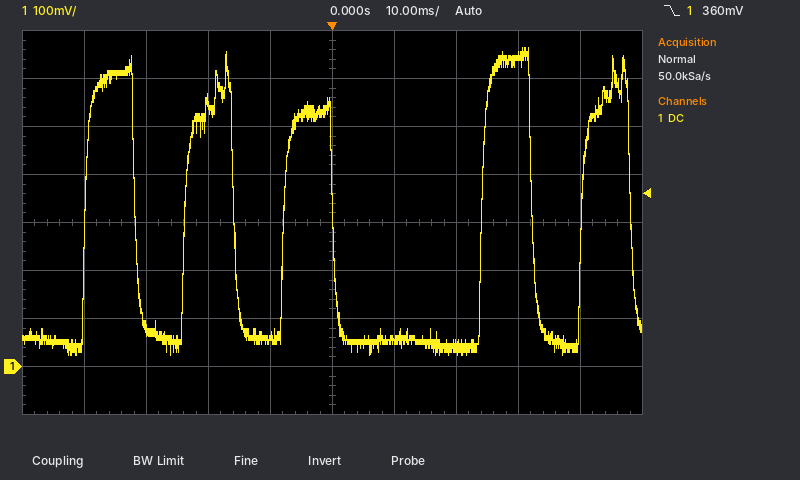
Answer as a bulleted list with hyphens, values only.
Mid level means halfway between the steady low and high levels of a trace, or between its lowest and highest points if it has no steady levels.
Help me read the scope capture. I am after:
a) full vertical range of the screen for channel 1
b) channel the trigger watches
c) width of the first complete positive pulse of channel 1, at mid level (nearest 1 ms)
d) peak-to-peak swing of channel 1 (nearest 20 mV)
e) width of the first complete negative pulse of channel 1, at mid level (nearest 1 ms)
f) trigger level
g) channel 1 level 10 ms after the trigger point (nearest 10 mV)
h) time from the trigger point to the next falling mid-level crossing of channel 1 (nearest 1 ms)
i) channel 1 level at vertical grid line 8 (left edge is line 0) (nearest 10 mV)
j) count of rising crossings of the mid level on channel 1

- 800 mV
- channel 1
- 8 ms
- 640 mV
- 8 ms
- 360 mV
- 60 mV
- 32 ms
- 650 mV
- 5
